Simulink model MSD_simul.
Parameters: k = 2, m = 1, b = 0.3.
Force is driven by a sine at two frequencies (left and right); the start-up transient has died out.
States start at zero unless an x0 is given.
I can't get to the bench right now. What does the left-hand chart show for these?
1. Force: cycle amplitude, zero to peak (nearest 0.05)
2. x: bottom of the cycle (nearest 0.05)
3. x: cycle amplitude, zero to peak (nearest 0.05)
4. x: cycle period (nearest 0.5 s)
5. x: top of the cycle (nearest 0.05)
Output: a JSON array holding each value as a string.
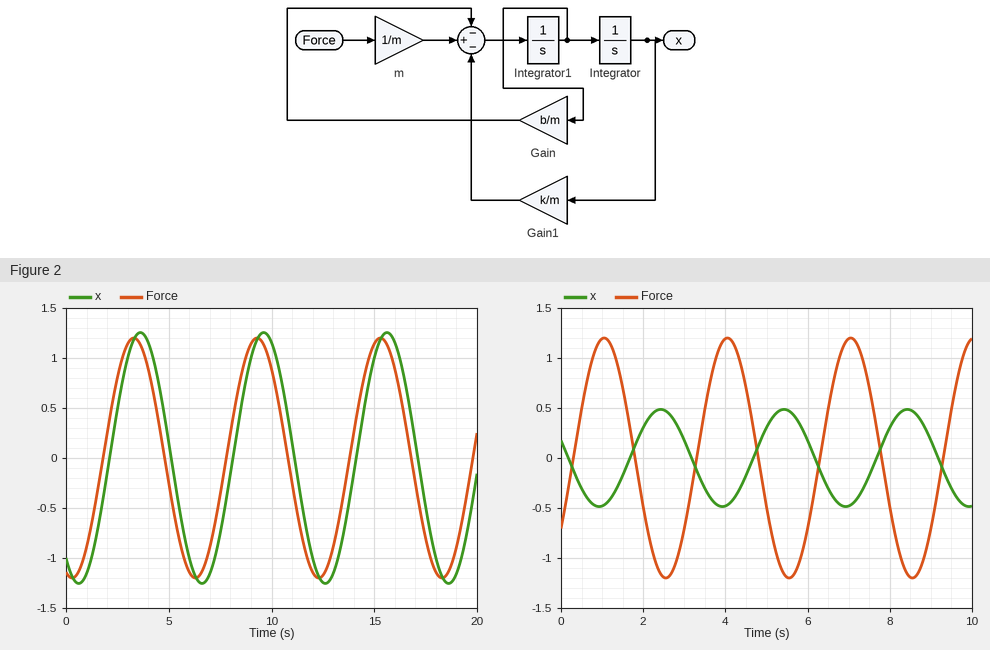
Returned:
["1.20", "-1.25", "1.25", "6.0 s", "1.25"]
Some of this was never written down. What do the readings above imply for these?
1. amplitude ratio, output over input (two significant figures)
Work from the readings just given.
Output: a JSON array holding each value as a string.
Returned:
["1.0"]
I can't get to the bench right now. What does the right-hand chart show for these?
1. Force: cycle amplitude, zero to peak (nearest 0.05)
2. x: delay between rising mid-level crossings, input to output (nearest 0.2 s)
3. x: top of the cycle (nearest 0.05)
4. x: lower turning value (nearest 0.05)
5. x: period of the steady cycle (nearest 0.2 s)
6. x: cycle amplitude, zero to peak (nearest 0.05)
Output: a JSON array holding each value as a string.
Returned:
["1.20", "1.4 s", "0.50", "-0.50", "3.0 s", "0.50"]
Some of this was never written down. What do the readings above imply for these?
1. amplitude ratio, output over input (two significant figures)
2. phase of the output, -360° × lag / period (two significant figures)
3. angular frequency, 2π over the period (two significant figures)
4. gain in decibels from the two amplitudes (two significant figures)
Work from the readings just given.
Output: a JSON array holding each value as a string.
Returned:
["0.42", "-170°", "2.1 rad/s", "-7.6 dB"]
